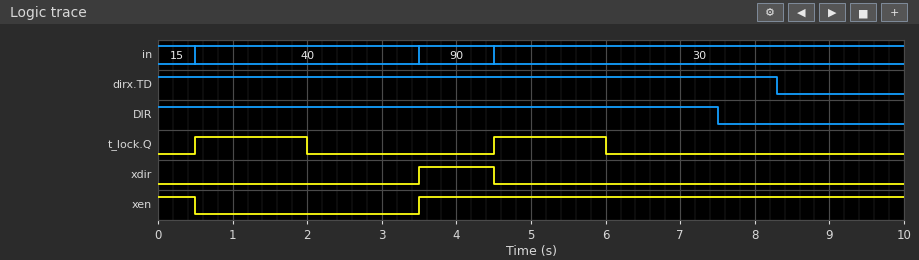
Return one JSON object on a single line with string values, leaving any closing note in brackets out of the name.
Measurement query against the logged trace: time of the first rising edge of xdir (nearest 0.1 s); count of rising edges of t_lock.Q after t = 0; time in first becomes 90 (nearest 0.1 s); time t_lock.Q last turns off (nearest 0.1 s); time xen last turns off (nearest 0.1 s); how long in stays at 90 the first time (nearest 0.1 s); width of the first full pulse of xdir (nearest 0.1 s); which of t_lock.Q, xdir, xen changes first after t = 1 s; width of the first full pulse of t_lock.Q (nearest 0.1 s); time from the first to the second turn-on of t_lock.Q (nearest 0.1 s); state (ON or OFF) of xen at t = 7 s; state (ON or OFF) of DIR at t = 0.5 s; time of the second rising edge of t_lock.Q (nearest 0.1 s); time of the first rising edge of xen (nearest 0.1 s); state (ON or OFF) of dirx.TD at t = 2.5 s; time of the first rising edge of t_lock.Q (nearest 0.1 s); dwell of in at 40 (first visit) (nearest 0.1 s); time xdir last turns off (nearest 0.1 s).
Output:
{"time of the first rising edge of xdir": "3.5 s", "count of rising edges of t_lock.Q after t = 0": "2", "time in first becomes 90": "3.5 s", "time t_lock.Q last turns off": "6.0 s", "time xen last turns off": "0.5 s", "how long in stays at 90 the first time": "1.0 s", "width of the first full pulse of xdir": "1.0 s", "which of t_lock.Q, xdir, xen changes first after t = 1 s": "t_lock.Q", "width of the first full pulse of t_lock.Q": "1.5 s", "time from the first to the second turn-on of t_lock.Q": "4.0 s", "state (ON or OFF) of xen at t = 7 s": "ON", "state (ON or OFF) of DIR at t = 0.5 s": "ON", "time of the second rising edge of t_lock.Q": "4.5 s", "time of the first rising edge of xen": "3.5 s", "state (ON or OFF) of dirx.TD at t = 2.5 s": "ON", "time of the first rising edge of t_lock.Q": "0.5 s", "dwell of in at 40 (first visit)": "3.0 s", "time xdir last turns off": "4.5 s"}
